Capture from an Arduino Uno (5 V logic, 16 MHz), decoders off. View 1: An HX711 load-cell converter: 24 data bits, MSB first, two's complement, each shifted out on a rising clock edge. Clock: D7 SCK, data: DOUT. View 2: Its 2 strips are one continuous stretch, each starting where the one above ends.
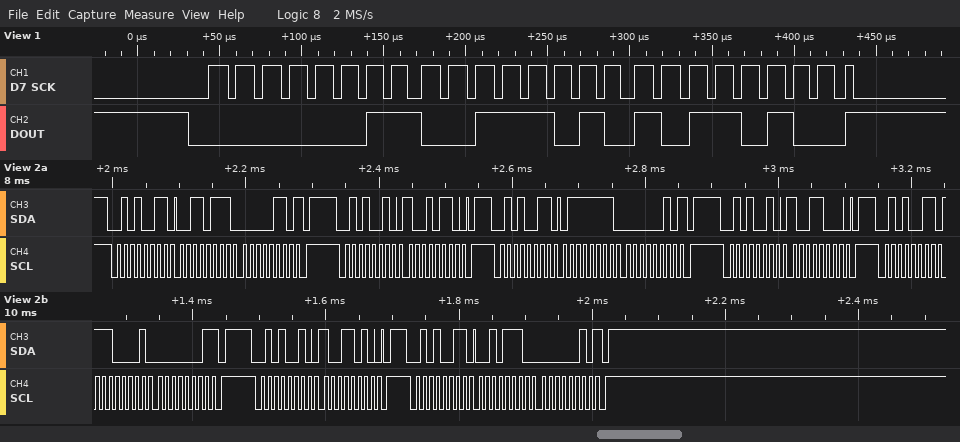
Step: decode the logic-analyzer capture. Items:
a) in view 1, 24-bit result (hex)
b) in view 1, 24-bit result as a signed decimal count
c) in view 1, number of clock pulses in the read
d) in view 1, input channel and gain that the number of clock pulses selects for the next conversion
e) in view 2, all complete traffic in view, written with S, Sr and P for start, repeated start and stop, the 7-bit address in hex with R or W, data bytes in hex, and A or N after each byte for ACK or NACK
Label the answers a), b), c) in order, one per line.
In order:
a) 0x033AB4
b) 211636
c) 25
d) channel A, gain 128
e) S 29R A 37 A 06 N P S 29W A 96 A P S 29R A 7F A 02 N P S 29W A 98 A P S 29R A E1 A 01 N P S 29W A 9A A P S 29R A 2E A 02 N P
